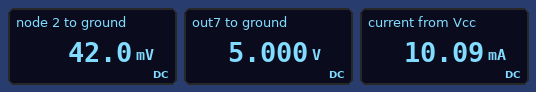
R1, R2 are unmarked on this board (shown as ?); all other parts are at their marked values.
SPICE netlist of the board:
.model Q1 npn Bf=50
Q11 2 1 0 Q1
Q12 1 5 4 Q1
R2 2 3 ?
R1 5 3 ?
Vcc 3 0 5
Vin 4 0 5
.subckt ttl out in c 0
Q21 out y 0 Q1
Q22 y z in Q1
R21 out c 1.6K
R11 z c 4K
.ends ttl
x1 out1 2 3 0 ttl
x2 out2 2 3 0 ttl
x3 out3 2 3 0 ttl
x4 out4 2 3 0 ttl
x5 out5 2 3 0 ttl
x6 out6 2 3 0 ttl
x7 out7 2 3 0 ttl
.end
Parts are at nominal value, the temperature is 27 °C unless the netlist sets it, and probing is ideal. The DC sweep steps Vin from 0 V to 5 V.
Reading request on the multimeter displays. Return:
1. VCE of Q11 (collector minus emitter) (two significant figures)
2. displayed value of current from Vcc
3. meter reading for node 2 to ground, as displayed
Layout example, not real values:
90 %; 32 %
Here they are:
42 mV; 10.09 mA; 42.0 mV
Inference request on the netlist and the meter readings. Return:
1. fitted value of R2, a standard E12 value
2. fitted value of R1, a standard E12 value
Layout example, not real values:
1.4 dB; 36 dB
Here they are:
3.9 kΩ; 2.2 kΩ
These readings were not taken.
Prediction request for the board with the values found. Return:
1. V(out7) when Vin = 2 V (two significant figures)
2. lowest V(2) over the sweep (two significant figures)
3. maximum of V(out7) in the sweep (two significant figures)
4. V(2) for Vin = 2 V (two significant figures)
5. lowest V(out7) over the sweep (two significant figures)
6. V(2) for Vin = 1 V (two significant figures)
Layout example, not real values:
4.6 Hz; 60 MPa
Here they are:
5.0 V; 42 mV; 5.0 V; 42 mV; 44 mV; 42 mV
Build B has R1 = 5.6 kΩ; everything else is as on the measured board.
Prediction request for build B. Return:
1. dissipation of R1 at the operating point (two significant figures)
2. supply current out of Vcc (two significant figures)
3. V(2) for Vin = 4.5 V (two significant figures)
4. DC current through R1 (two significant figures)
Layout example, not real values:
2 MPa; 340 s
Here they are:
2.1 mW; 9.1 mA; 61 mV; 610 µA
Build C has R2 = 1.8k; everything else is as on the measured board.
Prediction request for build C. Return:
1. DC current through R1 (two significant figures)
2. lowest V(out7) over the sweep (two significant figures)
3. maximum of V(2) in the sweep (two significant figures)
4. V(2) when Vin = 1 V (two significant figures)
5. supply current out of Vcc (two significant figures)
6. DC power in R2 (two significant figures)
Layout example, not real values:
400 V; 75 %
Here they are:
1.5 mA; 41 mV; 830 mV; 45 mV; 12 mA; 14 mW
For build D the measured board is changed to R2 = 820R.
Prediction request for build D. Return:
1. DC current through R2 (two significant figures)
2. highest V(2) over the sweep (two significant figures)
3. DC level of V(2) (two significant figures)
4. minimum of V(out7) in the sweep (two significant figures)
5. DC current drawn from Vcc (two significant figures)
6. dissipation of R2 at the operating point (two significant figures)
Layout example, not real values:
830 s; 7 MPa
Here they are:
6.0 mA; 870 mV; 50 mV; 37 mV; 15 mA; 30 mW
